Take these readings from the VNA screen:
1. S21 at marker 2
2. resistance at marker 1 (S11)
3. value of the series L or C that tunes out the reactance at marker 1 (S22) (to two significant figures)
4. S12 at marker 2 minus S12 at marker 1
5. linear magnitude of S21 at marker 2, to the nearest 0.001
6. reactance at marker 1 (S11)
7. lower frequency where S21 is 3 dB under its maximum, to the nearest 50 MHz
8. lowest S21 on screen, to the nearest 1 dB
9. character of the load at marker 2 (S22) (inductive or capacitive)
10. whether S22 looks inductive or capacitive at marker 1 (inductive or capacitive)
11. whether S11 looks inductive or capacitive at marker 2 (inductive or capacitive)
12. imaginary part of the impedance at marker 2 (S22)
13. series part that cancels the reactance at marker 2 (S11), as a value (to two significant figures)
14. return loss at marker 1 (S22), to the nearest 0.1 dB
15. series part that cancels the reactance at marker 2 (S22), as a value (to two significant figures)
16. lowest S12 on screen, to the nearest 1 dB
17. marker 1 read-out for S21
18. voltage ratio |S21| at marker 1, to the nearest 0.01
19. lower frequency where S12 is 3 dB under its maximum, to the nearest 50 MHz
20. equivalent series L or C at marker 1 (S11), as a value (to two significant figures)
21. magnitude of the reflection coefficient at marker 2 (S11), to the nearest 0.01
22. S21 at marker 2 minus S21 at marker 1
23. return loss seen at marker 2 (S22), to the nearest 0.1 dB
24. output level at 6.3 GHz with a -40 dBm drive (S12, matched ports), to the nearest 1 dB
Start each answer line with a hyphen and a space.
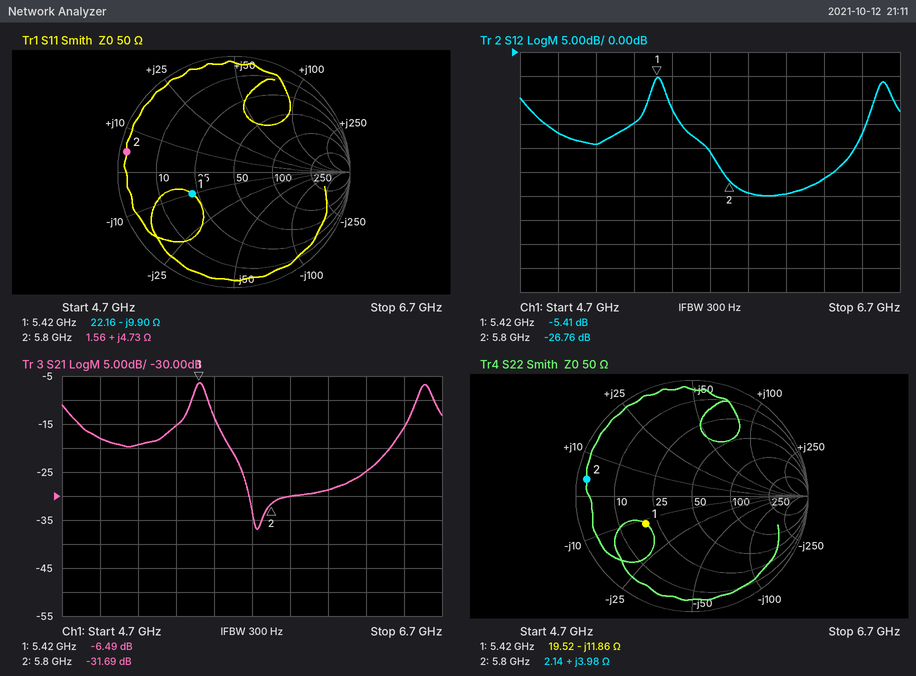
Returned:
- -31.69 dB
- 22.16 Ω
- 350 pH
- -21.35 dB
- 0.026
- -9.90 Ω
- 5.40 GHz
- -37 dB
- inductive
- capacitive
- inductive
- +3.98 Ω
- 5.8 pF
- 6.7 dB
- 6.9 pF
- -30 dB
- -6.49 dB
- 0.47
- 5.40 GHz
- 3.0 pF
- 0.94
- -25.20 dB
- 0.7 dB
- -66 dBm
